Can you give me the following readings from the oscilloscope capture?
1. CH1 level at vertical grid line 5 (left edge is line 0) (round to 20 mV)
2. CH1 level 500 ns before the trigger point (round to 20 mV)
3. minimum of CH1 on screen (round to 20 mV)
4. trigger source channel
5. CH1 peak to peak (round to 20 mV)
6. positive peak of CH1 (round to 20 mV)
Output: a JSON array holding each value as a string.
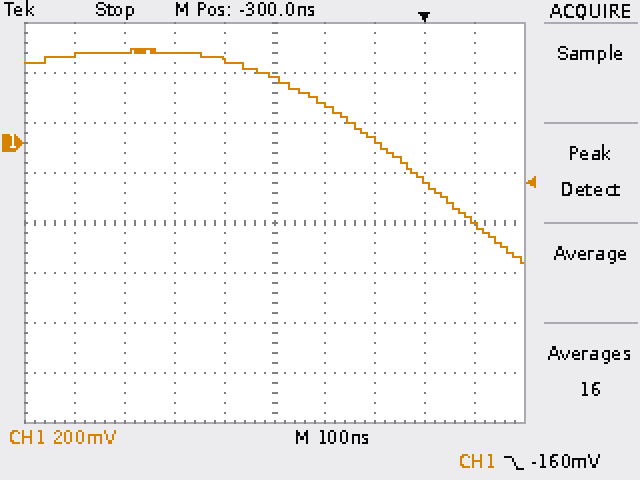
["260 mV", "360 mV", "-480 mV", "CH1", "860 mV", "380 mV"]
